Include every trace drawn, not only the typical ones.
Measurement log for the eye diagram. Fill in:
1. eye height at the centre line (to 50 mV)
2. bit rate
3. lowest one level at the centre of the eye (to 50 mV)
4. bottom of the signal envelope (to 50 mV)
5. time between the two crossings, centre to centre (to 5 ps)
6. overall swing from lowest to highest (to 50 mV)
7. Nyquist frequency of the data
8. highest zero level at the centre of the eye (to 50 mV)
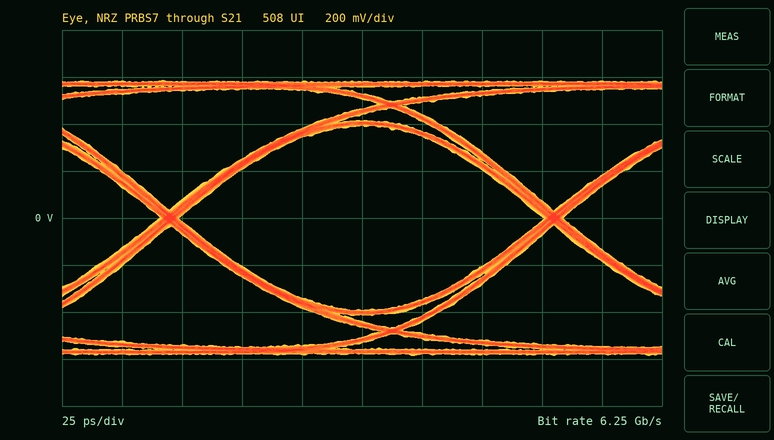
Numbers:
800 mV
6.25 Gb/s
400 mV
-600 mV
160 ps
1.15 V
3.125 GHz
-400 mV
